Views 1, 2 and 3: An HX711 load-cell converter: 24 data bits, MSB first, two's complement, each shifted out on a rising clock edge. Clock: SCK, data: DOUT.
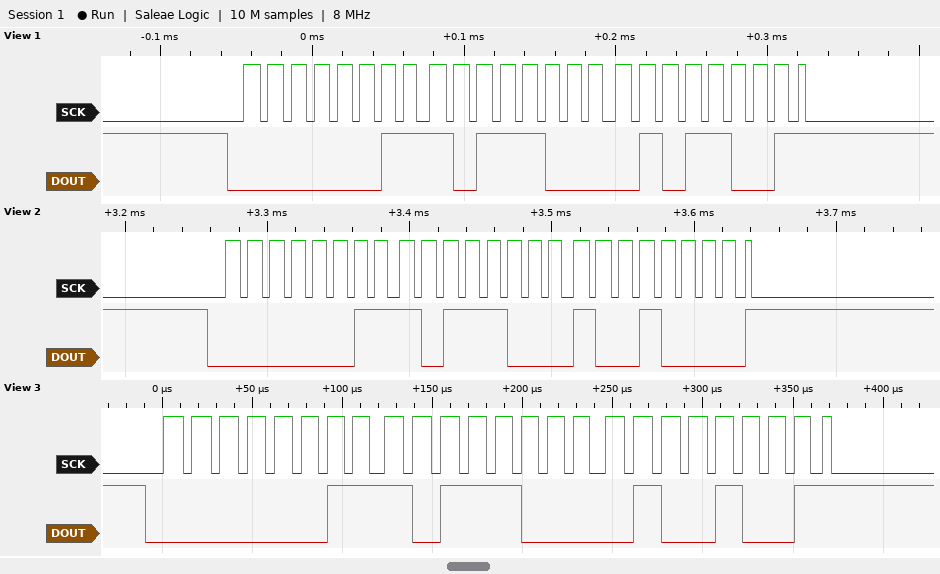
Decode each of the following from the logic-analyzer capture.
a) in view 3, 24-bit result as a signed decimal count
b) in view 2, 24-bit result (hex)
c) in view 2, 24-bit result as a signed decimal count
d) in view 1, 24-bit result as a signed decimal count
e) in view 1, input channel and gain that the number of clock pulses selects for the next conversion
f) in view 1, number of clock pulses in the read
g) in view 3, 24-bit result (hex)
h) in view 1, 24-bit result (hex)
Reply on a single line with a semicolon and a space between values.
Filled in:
243785; 0x03B890; 243856; 243801; channel A, gain 128; 25; 0x03B849; 0x03B859
